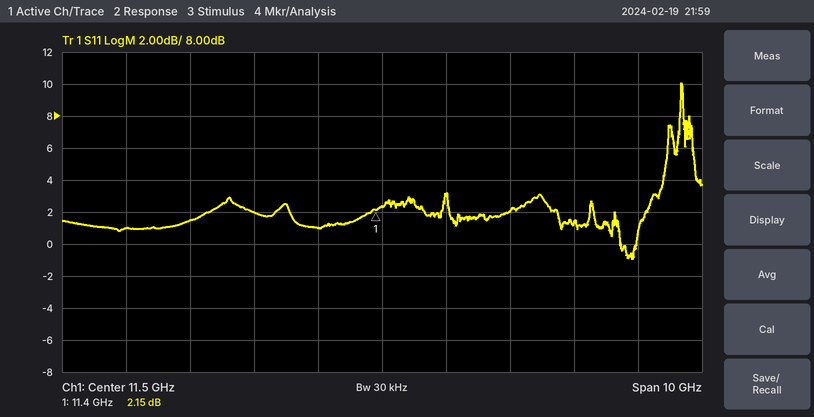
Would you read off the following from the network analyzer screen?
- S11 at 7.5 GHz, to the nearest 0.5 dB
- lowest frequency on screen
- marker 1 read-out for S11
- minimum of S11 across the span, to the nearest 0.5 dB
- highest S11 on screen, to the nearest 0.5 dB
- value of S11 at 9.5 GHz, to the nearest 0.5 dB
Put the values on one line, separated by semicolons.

1.0 dB; 6.5 GHz; 2.15 dB; -1.0 dB; 10.0 dB; 2.0 dB
